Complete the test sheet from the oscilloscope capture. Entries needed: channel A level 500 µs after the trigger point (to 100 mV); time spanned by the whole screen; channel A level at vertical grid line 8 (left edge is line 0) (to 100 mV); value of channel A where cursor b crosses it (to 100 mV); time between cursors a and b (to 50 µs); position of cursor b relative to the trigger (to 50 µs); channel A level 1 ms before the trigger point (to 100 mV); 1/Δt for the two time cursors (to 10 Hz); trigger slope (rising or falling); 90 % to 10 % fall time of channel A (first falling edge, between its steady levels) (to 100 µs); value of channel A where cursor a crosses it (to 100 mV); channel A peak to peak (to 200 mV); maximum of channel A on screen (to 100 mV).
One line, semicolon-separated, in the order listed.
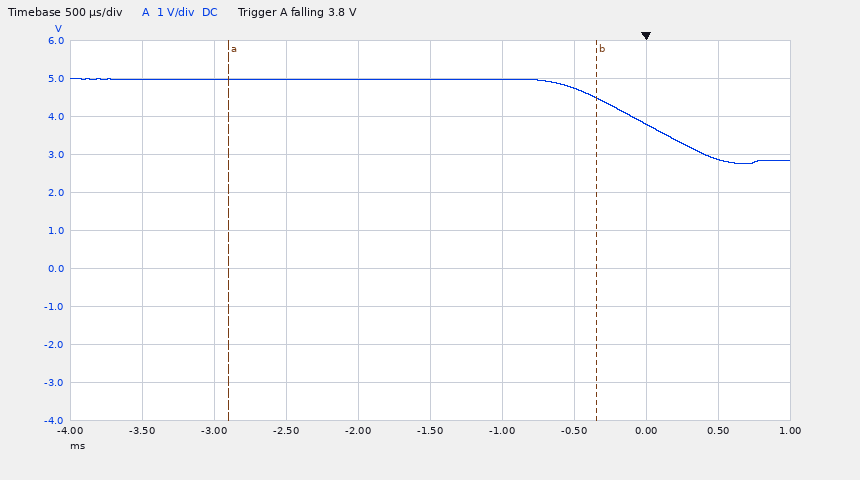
2.9 V; 5 ms; 3.8 V; 4.5 V; 2.55 ms; -350 µs; 5.0 V; 390 Hz; falling; 900 µs; 5.0 V; 2.2 V; 5.0 V
